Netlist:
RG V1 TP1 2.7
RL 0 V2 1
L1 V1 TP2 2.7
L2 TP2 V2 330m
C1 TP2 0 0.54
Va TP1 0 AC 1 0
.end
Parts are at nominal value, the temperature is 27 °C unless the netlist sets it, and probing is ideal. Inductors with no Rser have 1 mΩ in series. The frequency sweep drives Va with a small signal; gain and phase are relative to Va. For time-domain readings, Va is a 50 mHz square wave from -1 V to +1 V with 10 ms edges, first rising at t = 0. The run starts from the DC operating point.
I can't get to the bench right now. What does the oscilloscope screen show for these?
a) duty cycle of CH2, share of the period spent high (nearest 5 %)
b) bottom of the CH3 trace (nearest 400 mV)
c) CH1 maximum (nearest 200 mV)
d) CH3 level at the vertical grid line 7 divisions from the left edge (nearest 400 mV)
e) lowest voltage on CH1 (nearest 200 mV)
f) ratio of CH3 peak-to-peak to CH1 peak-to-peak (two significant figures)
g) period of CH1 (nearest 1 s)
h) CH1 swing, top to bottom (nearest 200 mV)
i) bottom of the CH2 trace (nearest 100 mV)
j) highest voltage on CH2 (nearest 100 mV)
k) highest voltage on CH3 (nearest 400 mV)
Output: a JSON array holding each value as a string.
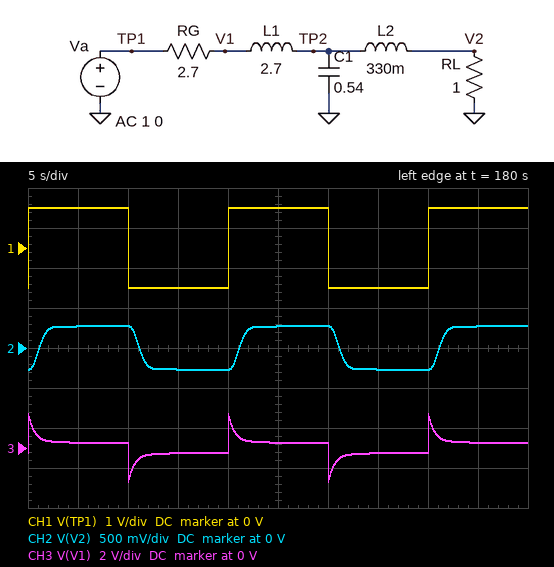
["50 %", "-1.6 V", "1.0 V", "-400 mV", "-1.0 V", "1.7", "20 s", "2.0 V", "-300 mV", "300 mV", "1.6 V"]
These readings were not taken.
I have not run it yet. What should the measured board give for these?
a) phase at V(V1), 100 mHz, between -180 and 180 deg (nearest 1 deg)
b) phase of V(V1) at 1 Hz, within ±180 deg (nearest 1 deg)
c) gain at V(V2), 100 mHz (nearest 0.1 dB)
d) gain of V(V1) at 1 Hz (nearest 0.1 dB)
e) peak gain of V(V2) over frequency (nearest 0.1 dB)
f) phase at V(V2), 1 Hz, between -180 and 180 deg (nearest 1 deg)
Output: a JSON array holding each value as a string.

["34 deg", "9 deg", "-12.0 dB", "-0.1 dB", "-11.4 dB", "129 deg"]
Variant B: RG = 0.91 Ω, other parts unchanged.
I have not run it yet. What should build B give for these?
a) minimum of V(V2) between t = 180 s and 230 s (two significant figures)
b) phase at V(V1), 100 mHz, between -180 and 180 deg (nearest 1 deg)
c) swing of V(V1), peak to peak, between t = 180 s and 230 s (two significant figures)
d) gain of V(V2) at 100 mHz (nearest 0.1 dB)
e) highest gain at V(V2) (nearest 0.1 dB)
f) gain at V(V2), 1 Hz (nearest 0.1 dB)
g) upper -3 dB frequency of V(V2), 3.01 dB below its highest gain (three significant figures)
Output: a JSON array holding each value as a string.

["-520 mV", "18 deg", "2.9 V", "-7.8 dB", "-5.6 dB", "-41.2 dB", "126 mHz"]
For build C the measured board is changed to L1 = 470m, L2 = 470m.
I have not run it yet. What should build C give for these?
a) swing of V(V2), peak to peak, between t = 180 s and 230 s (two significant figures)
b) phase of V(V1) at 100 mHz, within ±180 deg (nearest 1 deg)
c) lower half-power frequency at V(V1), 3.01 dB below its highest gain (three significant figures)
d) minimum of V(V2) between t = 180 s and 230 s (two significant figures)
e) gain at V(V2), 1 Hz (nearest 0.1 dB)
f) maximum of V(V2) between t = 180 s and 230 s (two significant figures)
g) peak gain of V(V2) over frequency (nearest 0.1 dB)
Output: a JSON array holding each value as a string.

["650 mV", "8 deg", "1.02 Hz", "-330 mV", "-31.2 dB", "330 mV", "-11.0 dB"]
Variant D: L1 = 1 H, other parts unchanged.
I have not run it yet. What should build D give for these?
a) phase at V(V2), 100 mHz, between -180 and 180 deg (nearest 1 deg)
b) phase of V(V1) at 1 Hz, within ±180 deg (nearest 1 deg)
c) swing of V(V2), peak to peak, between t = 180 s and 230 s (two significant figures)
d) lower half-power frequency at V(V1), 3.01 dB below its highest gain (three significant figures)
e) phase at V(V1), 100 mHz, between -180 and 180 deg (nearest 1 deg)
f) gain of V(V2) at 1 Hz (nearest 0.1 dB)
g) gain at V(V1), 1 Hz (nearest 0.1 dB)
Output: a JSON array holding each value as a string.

["-27 deg", "24 deg", "610 mV", "562 mHz", "18 deg", "-33.1 dB", "-0.8 dB"]
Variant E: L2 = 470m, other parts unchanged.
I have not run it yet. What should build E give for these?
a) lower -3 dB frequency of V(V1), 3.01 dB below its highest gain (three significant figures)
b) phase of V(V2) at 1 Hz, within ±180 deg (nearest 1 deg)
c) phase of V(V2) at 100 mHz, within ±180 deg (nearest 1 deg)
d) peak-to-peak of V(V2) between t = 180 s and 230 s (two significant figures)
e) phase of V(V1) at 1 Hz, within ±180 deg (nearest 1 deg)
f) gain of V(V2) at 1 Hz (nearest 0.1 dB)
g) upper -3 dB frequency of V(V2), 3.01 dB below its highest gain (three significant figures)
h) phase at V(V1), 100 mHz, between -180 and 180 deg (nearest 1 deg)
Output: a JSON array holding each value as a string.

["244 mHz", "120 deg", "-44 deg", "550 mV", "9 deg", "-44.2 dB", "276 mHz", "33 deg"]
